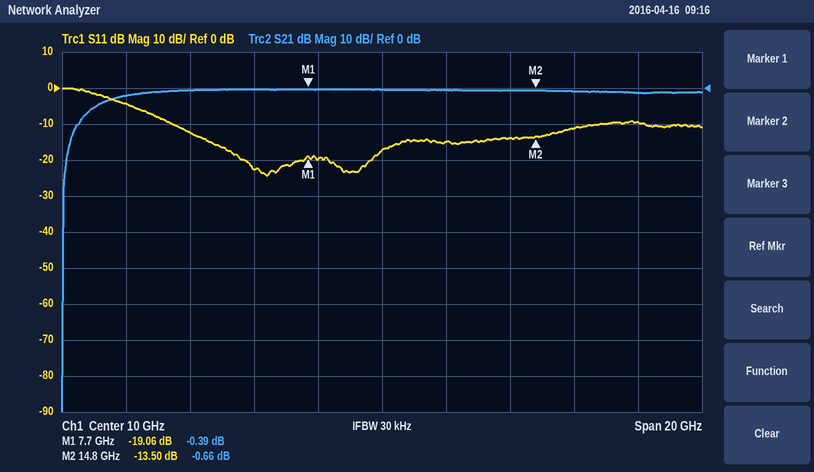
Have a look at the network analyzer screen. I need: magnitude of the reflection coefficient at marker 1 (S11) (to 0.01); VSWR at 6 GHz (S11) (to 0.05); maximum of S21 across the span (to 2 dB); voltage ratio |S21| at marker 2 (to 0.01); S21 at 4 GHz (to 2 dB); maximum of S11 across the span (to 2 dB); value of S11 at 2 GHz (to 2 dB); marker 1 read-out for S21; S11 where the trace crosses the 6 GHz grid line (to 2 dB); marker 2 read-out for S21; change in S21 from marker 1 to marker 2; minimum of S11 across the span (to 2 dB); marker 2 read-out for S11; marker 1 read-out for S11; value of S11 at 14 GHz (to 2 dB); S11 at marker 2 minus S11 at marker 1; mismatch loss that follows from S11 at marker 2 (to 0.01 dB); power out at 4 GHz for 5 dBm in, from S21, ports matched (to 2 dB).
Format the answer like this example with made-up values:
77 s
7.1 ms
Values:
0.11
1.15
0 dB
0.93
0 dB
0 dB
-4 dB
-0.39 dB
-22 dB
-0.66 dB
-0.27 dB
-24 dB
-13.50 dB
-19.06 dB
-14 dB
5.56 dB
0.20 dB
4 dBm
